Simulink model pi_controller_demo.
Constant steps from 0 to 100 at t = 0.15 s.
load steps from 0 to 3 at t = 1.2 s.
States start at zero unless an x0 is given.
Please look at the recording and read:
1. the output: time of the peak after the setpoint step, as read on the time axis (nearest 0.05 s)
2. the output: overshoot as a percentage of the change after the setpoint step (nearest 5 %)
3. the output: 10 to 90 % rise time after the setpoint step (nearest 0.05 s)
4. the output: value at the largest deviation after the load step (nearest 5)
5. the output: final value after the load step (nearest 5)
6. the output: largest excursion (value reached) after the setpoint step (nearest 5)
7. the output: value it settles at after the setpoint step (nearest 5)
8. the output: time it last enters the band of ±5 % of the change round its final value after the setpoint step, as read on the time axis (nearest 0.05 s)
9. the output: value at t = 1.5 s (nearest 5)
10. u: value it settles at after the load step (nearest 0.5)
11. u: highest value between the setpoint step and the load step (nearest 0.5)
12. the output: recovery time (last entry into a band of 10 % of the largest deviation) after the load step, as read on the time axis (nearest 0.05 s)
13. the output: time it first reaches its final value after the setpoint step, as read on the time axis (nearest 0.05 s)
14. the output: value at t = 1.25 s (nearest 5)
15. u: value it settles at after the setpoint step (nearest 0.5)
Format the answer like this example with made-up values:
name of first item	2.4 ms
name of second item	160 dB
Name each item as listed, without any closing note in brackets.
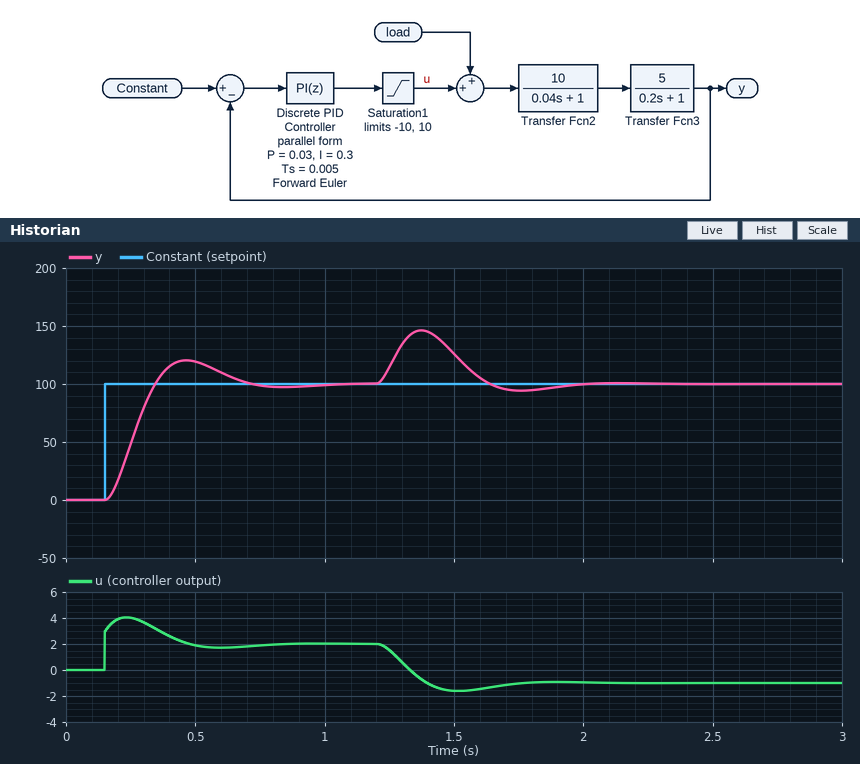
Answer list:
the output: time of the peak after the setpoint step, as read on the time axis	0.45 s
the output: overshoot as a percentage of the change after the setpoint step	20 %
the output: 10 to 90 % rise time after the setpoint step	0.15 s
the output: value at the largest deviation after the load step	145
the output: final value after the load step	100
the output: largest excursion (value reached) after the setpoint step	120
the output: value it settles at after the setpoint step	100
the output: time it last enters the band of ±5 % of the change round its final value after the setpoint step, as read on the time axis	0.65 s
the output: value at t = 1.5 s	125
u: value it settles at after the load step	-1.0
u: highest value between the setpoint step and the load step	4.0
the output: recovery time (last entry into a band of 10 % of the largest deviation) after the load step, as read on the time axis	1.85 s
the output: time it first reaches its final value after the setpoint step, as read on the time axis	0.35 s
the output: value at t = 1.25 s	115
u: value it settles at after the setpoint step	2.0
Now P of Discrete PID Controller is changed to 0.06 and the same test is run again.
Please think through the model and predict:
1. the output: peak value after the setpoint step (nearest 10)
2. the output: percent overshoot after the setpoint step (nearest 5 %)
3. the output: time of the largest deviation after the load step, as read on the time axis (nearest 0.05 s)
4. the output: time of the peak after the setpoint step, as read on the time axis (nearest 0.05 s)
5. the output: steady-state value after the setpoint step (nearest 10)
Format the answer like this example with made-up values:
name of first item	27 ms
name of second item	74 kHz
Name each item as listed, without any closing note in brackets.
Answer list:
the output: peak value after the setpoint step	110
the output: percent overshoot after the setpoint step	10 %
the output: time of the largest deviation after the load step, as read on the time axis	1.35 s
the output: time of the peak after the setpoint step, as read on the time axis	0.35 s
the output: steady-state value after the setpoint step	100
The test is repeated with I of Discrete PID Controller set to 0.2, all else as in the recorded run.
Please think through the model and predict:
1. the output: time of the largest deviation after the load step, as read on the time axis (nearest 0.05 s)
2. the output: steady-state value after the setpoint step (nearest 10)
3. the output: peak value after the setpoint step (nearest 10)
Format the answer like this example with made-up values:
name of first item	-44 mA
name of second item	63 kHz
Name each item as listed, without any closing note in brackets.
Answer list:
the output: time of the largest deviation after the load step, as read on the time axis	1.40 s
the output: steady-state value after the setpoint step	100
the output: peak value after the setpoint step	110
